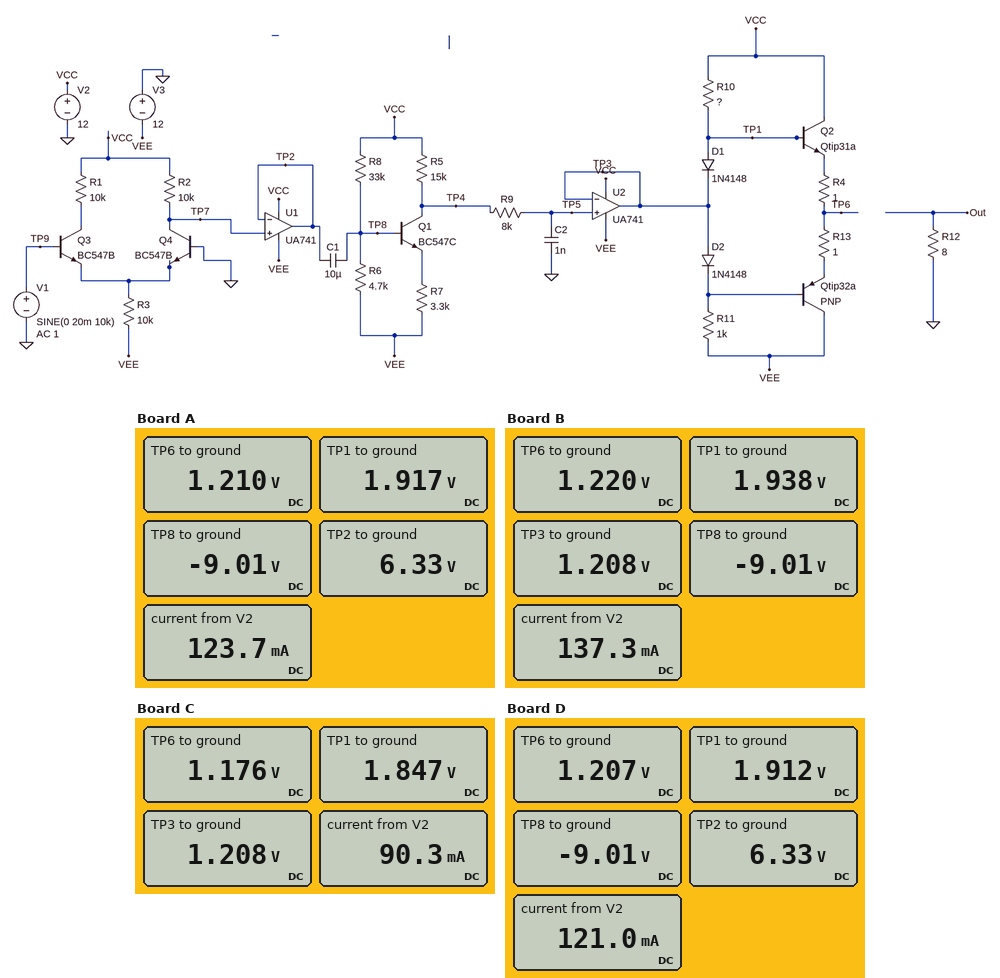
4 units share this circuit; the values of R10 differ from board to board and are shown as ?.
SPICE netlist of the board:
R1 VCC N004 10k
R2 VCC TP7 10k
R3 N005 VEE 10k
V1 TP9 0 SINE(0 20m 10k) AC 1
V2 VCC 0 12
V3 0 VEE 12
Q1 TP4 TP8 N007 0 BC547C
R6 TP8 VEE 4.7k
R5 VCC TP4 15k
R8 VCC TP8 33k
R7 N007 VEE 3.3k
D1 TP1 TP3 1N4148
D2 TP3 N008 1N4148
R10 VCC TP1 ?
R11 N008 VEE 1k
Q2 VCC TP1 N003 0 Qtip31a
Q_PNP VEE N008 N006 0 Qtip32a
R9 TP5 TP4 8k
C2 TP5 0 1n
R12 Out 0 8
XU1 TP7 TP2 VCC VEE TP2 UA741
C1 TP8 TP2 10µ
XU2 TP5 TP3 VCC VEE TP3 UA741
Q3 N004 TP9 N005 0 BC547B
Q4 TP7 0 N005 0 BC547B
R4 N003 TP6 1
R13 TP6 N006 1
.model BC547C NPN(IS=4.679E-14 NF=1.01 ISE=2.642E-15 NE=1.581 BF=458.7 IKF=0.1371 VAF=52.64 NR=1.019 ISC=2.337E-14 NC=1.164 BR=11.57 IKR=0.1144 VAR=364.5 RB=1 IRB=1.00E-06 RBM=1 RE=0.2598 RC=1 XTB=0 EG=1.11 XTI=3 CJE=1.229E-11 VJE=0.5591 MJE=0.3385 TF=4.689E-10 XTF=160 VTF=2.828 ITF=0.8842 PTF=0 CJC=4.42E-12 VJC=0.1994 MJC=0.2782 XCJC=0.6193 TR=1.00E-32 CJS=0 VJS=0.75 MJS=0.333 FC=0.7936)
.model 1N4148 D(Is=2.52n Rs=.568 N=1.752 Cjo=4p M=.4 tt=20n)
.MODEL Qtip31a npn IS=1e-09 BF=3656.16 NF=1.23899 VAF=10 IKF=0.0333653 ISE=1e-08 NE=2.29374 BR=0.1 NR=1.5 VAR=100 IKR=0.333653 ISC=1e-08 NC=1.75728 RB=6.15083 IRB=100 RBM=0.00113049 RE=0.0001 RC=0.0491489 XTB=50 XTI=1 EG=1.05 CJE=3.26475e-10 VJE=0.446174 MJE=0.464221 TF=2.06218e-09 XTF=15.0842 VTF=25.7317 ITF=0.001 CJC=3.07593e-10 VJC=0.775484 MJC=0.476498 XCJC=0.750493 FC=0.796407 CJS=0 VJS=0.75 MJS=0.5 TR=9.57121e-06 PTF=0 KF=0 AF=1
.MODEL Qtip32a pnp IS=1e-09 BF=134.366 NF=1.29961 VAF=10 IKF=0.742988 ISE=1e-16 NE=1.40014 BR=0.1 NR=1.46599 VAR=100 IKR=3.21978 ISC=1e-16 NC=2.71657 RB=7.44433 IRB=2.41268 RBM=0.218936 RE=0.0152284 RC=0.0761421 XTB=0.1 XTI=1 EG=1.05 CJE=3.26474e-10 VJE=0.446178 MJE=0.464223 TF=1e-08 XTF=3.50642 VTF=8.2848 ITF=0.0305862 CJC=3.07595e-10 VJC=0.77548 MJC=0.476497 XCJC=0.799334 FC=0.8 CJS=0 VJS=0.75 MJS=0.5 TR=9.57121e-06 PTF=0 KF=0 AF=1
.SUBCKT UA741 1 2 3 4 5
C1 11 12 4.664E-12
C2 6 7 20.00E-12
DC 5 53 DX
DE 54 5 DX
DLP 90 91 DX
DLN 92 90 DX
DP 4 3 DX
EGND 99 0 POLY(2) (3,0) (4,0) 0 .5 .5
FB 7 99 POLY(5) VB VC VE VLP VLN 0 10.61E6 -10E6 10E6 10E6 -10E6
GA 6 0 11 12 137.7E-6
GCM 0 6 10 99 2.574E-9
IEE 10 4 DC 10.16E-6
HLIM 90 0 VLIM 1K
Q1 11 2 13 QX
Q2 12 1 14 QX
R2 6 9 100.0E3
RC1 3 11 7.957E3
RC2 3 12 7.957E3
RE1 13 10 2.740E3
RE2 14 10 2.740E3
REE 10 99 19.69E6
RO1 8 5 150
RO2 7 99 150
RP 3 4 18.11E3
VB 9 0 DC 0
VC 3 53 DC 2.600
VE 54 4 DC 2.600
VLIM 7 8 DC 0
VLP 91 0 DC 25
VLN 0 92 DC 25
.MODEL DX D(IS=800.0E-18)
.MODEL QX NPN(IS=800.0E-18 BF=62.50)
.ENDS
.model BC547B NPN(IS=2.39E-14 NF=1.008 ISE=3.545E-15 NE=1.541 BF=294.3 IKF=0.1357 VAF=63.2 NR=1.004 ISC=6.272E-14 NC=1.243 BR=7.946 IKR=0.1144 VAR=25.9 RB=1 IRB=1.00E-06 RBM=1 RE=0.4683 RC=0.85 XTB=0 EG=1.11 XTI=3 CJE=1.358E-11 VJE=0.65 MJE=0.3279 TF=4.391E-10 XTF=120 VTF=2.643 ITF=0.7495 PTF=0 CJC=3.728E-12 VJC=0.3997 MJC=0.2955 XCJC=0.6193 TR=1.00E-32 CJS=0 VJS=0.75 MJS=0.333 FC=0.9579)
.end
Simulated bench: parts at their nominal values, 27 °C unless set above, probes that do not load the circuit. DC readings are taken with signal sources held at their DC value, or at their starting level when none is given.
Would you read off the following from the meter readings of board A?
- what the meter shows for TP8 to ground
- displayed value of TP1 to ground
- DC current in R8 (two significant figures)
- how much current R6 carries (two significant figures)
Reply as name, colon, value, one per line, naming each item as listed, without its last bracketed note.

what the meter shows for TP8 to ground: -9.01 V
displayed value of TP1 to ground: 1.917 V
DC current in R8: 640 µA
how much current R6 carries: 640 µA
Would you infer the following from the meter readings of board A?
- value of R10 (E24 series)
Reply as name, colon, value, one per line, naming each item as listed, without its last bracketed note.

value of R10: 750 Ω
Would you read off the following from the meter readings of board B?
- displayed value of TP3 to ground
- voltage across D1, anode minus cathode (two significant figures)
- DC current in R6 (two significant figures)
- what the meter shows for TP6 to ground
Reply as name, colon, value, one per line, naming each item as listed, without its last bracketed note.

displayed value of TP3 to ground: 1.208 V
voltage across D1, anode minus cathode: 730 mV
DC current in R6: 640 µA
what the meter shows for TP6 to ground: 1.220 V
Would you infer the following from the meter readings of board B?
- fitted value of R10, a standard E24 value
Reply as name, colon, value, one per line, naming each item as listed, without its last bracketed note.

fitted value of R10, a standard E24 value: 510 Ω
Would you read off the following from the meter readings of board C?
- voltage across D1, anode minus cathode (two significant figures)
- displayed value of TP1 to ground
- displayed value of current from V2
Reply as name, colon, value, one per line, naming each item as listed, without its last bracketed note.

voltage across D1, anode minus cathode: 640 mV
displayed value of TP1 to ground: 1.847 V
displayed value of current from V2: 90.3 mA
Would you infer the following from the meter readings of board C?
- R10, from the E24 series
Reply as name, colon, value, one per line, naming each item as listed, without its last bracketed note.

R10, from the E24 series: 3 kΩ
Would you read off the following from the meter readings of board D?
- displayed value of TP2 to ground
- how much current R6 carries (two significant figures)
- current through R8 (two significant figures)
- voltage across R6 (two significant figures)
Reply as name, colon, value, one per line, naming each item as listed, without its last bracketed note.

displayed value of TP2 to ground: 6.33 V
how much current R6 carries: 640 µA
current through R8: 640 µA
voltage across R6: 3.0 V
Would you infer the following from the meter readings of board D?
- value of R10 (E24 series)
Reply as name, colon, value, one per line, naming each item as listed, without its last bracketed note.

value of R10: 820 Ω
